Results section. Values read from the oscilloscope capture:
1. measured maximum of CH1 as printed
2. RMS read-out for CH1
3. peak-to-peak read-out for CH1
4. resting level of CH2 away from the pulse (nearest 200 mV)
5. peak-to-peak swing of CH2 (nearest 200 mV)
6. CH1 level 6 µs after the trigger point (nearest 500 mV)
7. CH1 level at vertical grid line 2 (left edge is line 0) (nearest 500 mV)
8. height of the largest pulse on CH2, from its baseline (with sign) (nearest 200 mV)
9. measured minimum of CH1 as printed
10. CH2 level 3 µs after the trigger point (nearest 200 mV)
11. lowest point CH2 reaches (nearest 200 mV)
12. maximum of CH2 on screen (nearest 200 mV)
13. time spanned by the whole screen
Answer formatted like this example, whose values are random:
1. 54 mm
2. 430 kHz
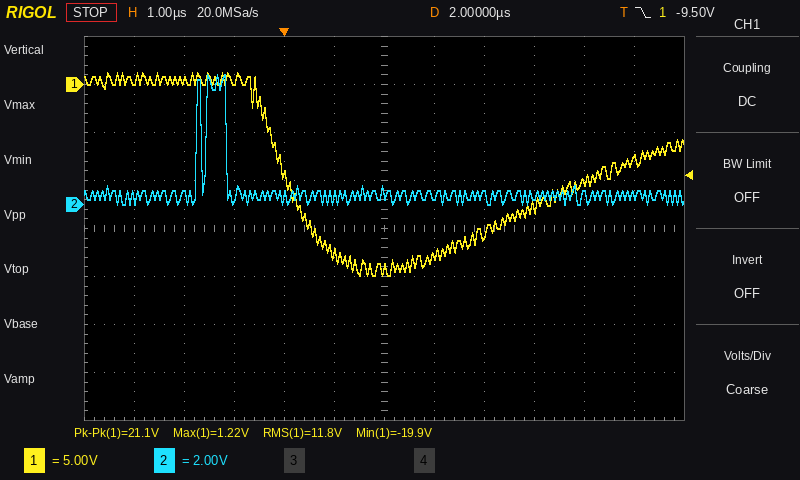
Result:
1. 1.22 V
2. 11.8 V
3. 21.1 V
4. 400 mV
5. 5.4 V
6. -10.0 V
7. 500 mV
8. +5.0 V
9. -19.9 V
10. 400 mV
11. 0.0 V
12. 5.4 V
13. 12 µs
